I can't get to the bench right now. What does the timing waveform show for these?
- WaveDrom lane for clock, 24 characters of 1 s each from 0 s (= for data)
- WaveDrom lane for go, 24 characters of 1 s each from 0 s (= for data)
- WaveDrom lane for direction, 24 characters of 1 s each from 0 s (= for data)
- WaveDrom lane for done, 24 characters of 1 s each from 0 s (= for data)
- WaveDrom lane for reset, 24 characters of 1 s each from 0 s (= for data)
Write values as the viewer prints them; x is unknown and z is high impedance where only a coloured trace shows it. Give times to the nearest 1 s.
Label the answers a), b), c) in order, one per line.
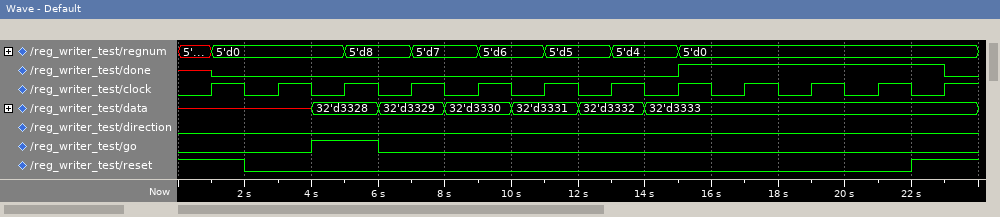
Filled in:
a) {name: 'clock', wave: '010101010101010101010101'}
b) {name: 'go', wave: '0...1.0.................'}
c) {name: 'direction', wave: '0.......................'}
d) {name: 'done', wave: 'x0.............1.......0'}
e) {name: 'reset', wave: '1.0...................1.'}
